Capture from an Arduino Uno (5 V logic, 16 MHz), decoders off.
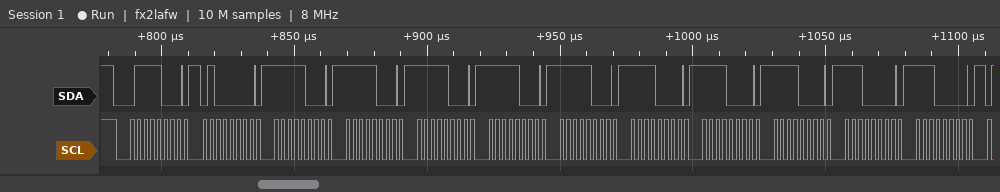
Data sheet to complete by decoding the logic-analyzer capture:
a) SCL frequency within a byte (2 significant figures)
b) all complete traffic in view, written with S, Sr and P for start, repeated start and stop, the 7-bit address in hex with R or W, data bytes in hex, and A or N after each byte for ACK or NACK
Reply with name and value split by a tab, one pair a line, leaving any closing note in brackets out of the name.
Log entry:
SCL frequency within a byte	400 kHz
all complete traffic in view, written with S, Sr and P for start, repeated start and stop, the 7-bit address in hex with R or W, data bytes in hex, and A or N after each byte for ACK or NACK	S 3CW A 40 A F8 A F8 A F8 A F8 A F8 A F0 A F0 A F0 A E0 A E0 A
